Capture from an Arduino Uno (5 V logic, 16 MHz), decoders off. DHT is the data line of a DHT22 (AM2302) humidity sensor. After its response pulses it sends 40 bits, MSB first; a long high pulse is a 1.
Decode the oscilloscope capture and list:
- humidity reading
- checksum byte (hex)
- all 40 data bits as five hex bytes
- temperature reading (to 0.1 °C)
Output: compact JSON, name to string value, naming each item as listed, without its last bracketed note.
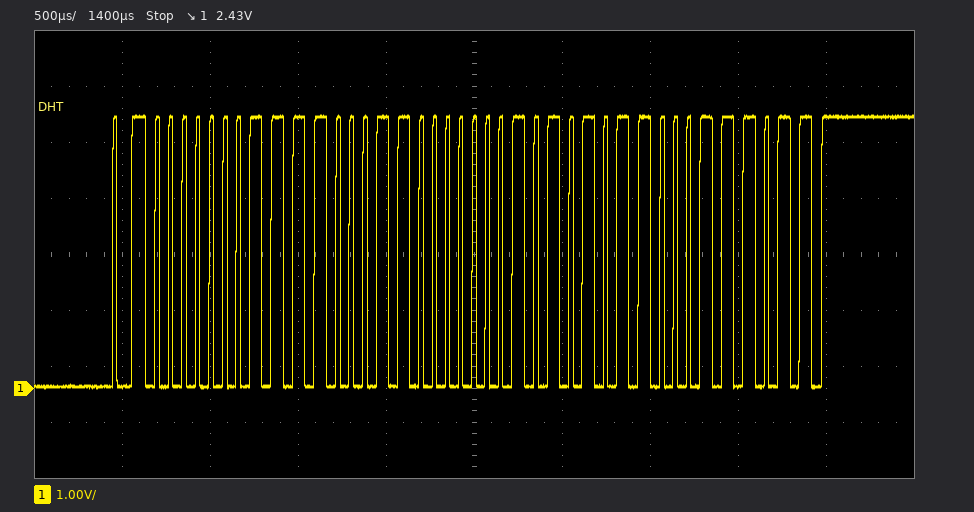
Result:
{"humidity reading": "48.3 %", "checksum byte": "0x3B", "all 40 data bits as five hex bytes": "01 E3 01 56 3B", "temperature reading": "34.2 °C"}
